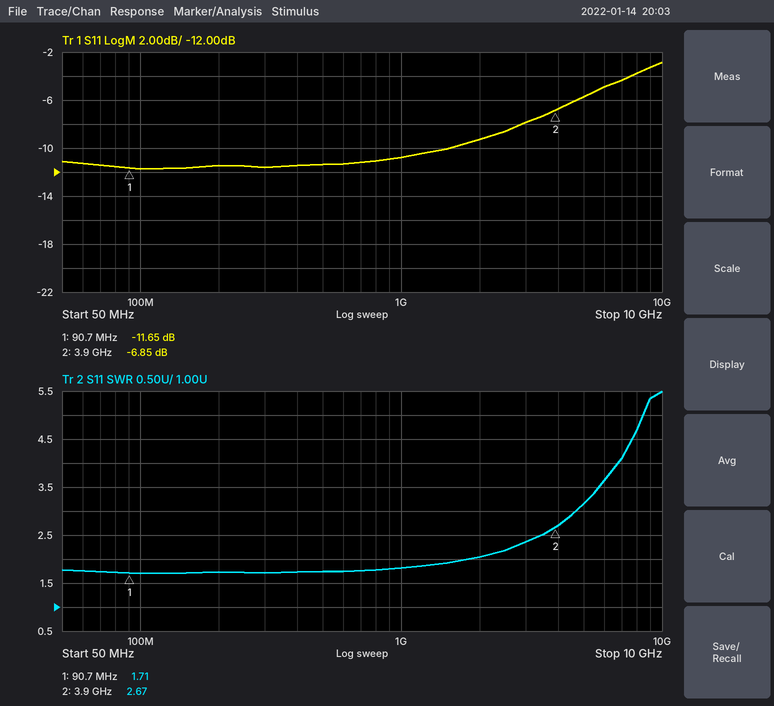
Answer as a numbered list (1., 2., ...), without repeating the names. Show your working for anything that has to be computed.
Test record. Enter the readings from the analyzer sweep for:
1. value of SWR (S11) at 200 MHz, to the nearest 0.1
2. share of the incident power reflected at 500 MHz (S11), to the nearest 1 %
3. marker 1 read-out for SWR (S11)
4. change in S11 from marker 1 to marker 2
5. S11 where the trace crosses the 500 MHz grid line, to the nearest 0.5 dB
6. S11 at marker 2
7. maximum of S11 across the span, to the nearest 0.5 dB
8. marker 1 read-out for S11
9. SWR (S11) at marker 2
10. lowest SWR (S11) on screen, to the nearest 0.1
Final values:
1. 1.7
2. 10^(-11.5/10) ≈ 7 %
3. 1.71
4. -6.85 − (-11.65) = 4.80 dB
5. -11.5 dB
6. -6.85 dB
7. -3.0 dB
8. -11.65 dB
9. 2.67
10. 1.7
